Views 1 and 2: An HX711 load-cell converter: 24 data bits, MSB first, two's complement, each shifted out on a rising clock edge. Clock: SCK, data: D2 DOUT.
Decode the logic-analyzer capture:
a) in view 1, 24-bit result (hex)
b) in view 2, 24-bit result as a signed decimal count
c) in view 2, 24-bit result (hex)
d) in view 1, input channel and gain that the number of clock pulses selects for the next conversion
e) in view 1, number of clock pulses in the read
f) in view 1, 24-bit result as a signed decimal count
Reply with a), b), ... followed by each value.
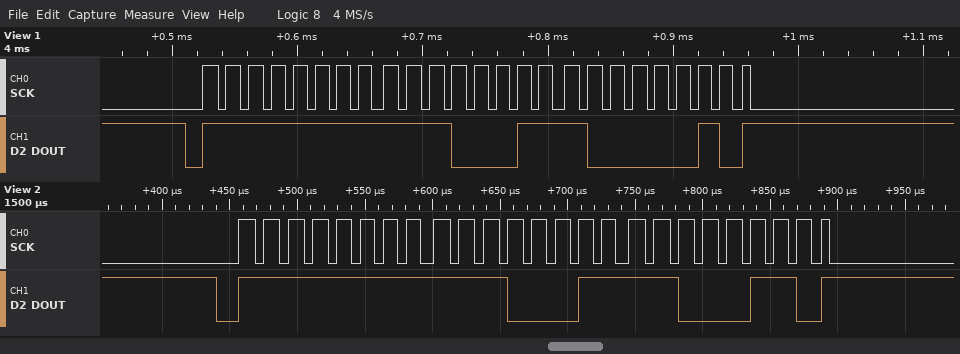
a) 0xFFE382
b) -7226
c) 0xFFE3C6
d) channel A, gain 128
e) 25
f) -7294
